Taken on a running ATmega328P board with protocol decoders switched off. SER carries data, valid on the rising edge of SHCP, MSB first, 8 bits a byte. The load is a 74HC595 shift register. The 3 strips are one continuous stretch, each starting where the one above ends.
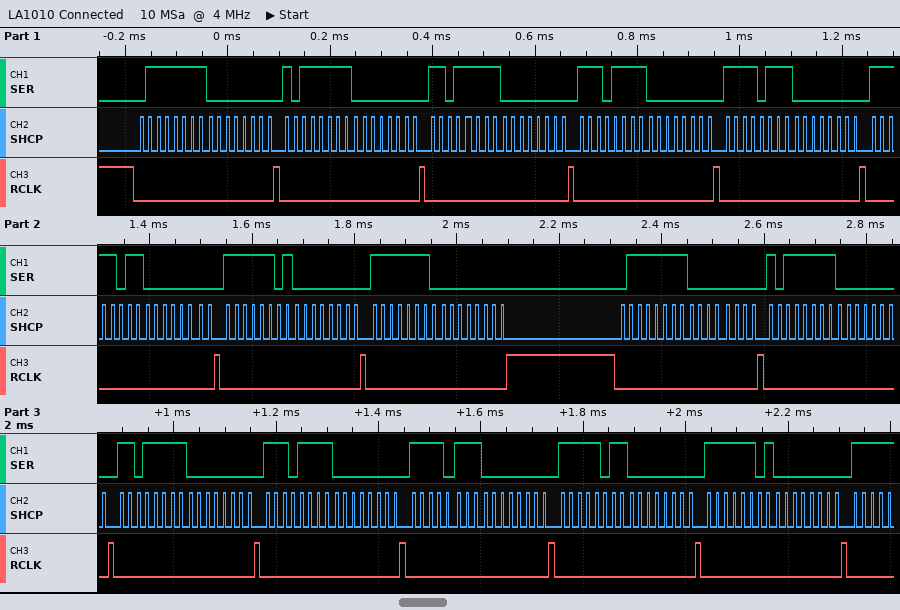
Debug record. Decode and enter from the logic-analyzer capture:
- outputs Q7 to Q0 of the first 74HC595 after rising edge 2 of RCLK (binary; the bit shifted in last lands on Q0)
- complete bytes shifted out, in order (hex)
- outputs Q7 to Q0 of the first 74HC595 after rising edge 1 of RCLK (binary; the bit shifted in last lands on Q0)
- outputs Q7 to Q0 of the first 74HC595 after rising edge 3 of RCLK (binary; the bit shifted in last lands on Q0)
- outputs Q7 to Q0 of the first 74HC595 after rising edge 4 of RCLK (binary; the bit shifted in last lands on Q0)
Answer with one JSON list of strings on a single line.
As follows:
["00000000", "7F 00 BF 00 DF 00 EF 00 F7 00 FB 00 FD 00 FE 00 7F 00 BF 00 DF 00 EF 00 F7 00 FB 00 FD 00", "00000000", "00000000", "00000000"]
